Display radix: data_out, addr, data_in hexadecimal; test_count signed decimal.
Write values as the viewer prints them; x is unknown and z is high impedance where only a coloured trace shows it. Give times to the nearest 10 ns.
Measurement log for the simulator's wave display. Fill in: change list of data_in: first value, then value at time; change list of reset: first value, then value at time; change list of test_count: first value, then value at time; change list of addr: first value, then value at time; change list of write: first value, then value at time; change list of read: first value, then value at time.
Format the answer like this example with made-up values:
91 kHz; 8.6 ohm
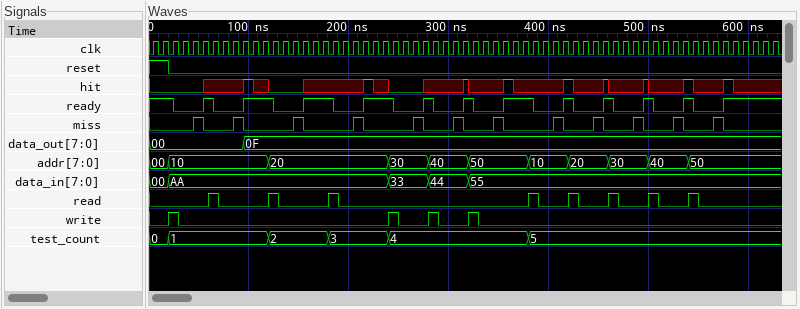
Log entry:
00, AA at 20 ns, 33 at 240 ns, 44 at 280 ns, 55 at 320 ns; 1, 0 at 20 ns; 0, 1 at 20 ns, 2 at 120 ns, 3 at 180 ns, 4 at 240 ns, 5 at 380 ns; 00, 10 at 20 ns, 20 at 120 ns, 30 at 240 ns, 40 at 280 ns, 50 at 320 ns, 10 at 380 ns, 20 at 420 ns, 30 at 460 ns, 40 at 500 ns, 50 at 540 ns; 0, 1 at 20 ns, 0 at 30 ns, 1 at 240 ns, 0 at 250 ns, 1 at 280 ns, 0 at 290 ns, 1 at 320 ns, 0 at 330 ns; 0, 1 at 60 ns, 0 at 70 ns, 1 at 120 ns, 0 at 130 ns, 1 at 180 ns, 0 at 190 ns, 1 at 380 ns, 0 at 390 ns, 1 at 420 ns, 0 at 430 ns, 1 at 460 ns, 0 at 470 ns, 1 at 500 ns, 0 at 510 ns, 1 at 540 ns, 0 at 550 ns
